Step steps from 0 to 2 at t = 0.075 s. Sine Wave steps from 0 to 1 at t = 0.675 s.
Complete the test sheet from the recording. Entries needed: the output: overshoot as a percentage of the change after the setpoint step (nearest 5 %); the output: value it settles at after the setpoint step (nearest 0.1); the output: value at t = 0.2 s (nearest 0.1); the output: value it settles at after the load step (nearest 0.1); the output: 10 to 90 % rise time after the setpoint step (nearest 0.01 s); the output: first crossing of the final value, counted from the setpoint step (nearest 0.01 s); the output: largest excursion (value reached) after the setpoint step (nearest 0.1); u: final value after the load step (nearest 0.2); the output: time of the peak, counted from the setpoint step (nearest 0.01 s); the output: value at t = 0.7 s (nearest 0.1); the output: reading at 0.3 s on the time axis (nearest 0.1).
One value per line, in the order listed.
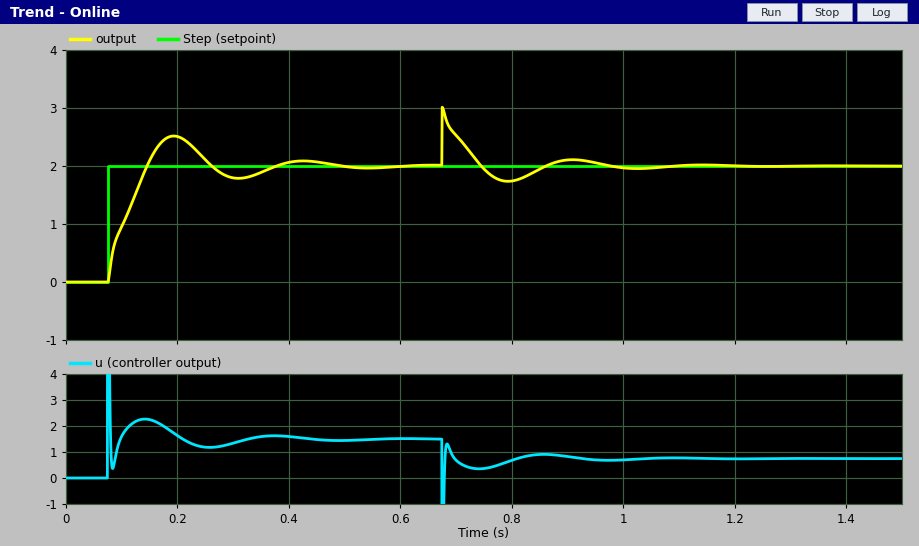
25 %
2.0
2.5
2.0
0.06 s
0.07 s
2.5
0.8
0.12 s
2.5
1.8
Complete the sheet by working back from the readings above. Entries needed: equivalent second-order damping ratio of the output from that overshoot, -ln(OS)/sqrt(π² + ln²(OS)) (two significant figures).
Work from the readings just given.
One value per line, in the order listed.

0.40
